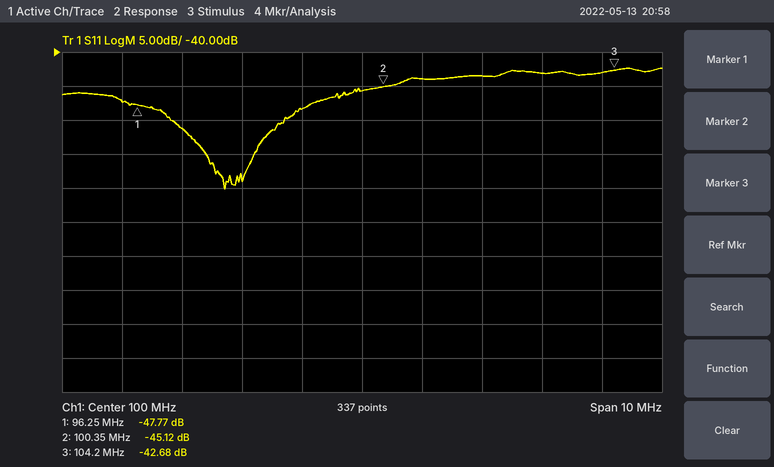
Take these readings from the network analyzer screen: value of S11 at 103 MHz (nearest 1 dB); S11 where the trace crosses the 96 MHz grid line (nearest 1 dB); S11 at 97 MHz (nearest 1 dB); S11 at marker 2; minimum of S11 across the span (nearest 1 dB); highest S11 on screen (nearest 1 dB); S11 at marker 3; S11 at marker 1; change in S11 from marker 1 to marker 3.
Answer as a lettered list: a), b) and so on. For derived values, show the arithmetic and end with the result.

a) -43 dB
b) -47 dB
c) -51 dB
d) -45.12 dB
e) -60 dB
f) -42 dB
g) -42.68 dB
h) -47.77 dB
i) -42.68 − (-47.77) = 5.09 dB
